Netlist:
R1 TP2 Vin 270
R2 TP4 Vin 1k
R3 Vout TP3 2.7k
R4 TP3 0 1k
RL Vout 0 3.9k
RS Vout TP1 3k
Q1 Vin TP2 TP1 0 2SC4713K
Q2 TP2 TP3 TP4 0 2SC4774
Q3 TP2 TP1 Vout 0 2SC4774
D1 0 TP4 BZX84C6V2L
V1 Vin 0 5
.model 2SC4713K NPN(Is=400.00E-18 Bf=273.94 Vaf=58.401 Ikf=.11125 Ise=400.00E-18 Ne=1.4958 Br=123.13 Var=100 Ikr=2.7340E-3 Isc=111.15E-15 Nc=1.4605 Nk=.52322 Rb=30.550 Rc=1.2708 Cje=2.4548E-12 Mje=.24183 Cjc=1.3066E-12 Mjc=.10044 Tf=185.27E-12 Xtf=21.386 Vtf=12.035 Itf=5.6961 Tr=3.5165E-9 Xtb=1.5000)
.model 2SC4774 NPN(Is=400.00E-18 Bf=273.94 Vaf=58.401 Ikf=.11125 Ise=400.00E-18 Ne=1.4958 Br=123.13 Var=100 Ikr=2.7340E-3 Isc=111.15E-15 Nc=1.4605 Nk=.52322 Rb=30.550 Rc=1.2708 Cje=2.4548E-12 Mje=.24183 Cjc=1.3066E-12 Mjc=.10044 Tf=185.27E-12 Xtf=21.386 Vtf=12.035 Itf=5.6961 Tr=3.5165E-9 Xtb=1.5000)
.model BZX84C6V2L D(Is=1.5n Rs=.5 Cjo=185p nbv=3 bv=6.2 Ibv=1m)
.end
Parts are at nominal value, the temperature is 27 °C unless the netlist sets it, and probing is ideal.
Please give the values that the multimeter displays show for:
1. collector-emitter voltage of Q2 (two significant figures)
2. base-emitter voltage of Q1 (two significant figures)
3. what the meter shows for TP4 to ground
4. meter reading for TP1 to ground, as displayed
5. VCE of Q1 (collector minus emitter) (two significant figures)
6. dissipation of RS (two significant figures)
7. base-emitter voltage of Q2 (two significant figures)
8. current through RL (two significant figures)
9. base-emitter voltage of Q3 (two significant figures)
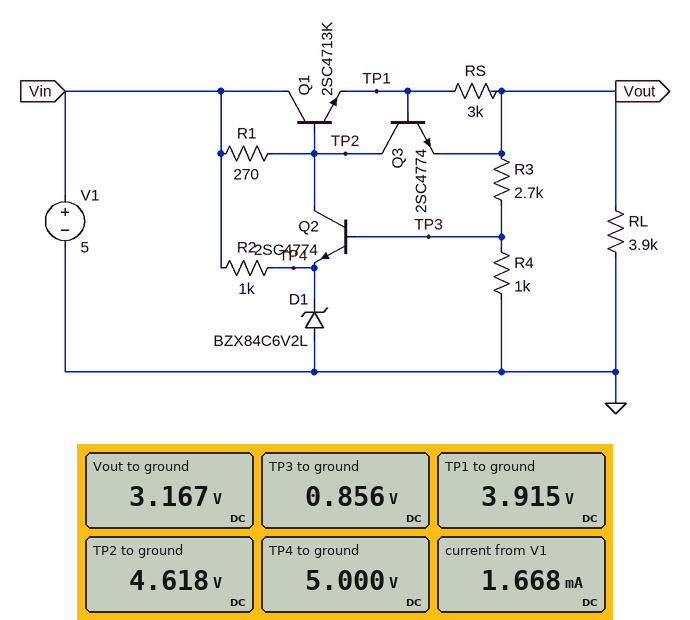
-380 mV
700 mV
5.000 V
3.915 V
1.1 V
190 µW
-4.1 V
810 µA
750 mV
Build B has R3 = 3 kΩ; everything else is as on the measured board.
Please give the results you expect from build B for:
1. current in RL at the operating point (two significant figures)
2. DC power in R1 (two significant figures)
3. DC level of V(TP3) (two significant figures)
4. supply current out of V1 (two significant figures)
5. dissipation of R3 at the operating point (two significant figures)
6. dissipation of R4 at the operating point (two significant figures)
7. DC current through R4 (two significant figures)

820 µA
500 µW
800 mV
1.6 mA
1.9 mW
630 µW
800 µA
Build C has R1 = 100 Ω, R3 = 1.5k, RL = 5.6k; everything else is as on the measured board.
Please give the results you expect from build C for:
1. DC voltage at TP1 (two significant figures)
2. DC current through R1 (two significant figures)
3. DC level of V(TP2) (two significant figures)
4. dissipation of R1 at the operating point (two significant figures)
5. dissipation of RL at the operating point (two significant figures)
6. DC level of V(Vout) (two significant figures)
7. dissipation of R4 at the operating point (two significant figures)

4.1 V
1.7 mA
4.8 V
290 µW
2.0 mW
3.4 V
1.8 mW
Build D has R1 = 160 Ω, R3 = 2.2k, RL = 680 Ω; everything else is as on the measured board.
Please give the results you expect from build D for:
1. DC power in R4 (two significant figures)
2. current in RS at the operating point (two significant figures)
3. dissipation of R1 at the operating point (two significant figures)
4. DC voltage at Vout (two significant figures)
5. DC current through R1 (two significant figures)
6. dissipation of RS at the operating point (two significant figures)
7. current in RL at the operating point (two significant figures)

750 µW
260 µA
3.5 mW
2.8 V
4.7 mA
200 µW
4.1 mA
